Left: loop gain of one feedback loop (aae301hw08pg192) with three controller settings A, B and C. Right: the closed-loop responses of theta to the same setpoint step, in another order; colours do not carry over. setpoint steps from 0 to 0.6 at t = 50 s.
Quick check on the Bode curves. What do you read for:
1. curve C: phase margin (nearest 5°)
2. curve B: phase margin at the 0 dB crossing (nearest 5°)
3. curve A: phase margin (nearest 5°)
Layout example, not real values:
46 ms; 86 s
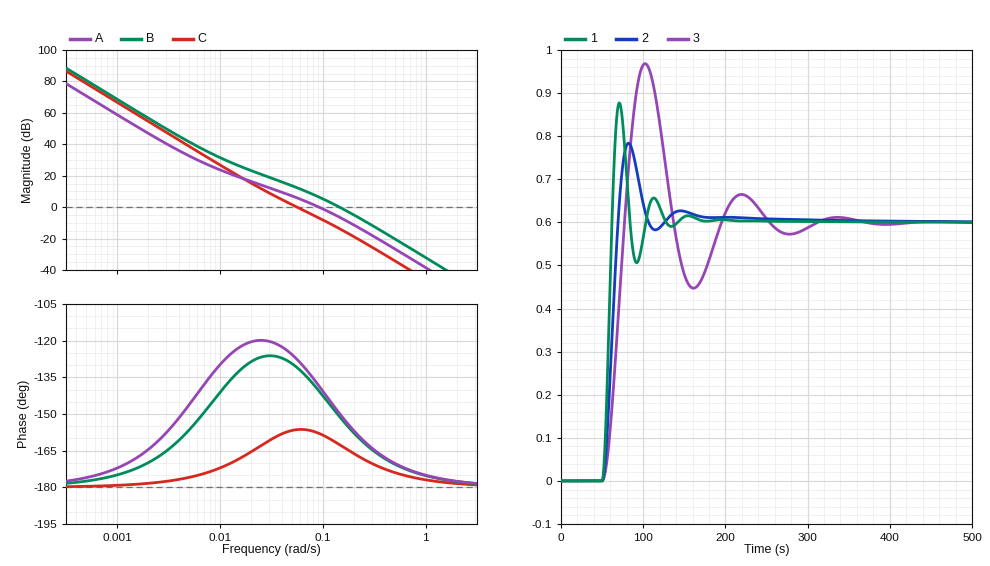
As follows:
25°; 30°; 40°
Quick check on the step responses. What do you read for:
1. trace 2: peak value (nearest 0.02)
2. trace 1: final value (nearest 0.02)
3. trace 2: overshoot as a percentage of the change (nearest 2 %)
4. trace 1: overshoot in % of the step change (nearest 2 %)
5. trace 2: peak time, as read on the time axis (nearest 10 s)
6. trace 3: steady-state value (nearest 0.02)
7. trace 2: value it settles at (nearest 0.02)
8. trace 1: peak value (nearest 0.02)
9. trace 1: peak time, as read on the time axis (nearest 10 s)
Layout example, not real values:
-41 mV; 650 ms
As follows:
0.78; 0.60; 30 %; 46 %; 80 s; 0.60; 0.60; 0.88; 70 s
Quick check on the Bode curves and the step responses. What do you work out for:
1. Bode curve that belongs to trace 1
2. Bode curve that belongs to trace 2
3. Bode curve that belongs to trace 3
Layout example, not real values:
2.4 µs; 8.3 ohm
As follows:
B; A; C
